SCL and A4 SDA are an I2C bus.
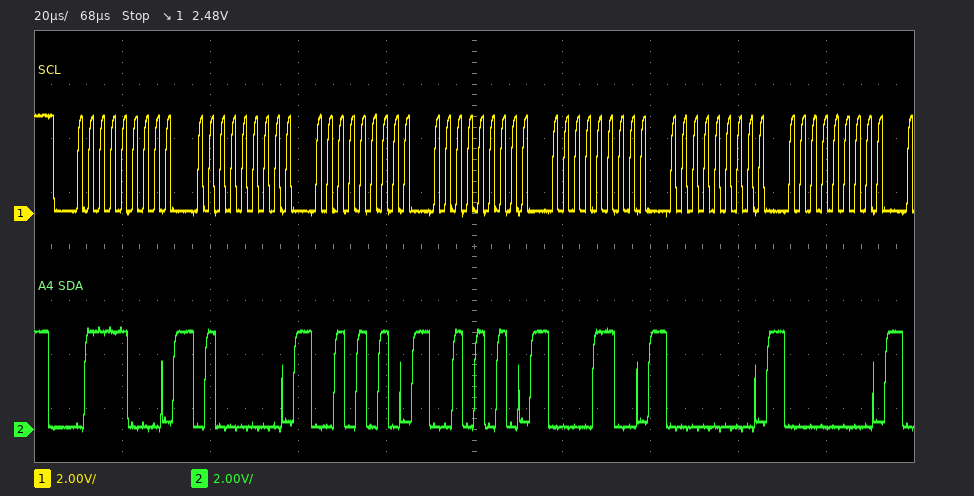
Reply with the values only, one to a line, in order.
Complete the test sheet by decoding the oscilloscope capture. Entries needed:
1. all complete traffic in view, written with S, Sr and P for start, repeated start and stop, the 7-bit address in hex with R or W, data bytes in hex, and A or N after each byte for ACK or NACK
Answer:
S 3CW A 40 A 2A A 2A A 0C A 00 A 00 A
